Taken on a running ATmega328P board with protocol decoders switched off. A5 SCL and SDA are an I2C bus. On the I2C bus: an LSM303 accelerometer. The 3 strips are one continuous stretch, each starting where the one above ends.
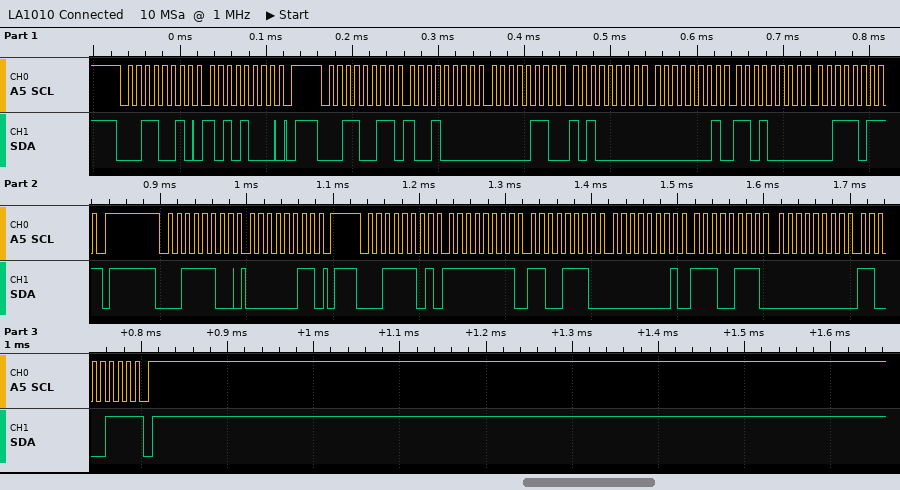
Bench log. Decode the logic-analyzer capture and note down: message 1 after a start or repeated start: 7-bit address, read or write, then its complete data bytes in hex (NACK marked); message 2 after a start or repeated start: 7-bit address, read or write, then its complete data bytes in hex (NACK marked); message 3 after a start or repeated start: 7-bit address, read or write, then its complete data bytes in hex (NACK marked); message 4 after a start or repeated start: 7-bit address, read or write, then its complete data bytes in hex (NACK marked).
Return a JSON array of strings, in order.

["0x19 write: A8", "0x19 read: 90 06 A0 01 D0 3B NACK", "0x1E write: 03", "0x1E read: FF CE 01 E7 00 C7 NACK"]
